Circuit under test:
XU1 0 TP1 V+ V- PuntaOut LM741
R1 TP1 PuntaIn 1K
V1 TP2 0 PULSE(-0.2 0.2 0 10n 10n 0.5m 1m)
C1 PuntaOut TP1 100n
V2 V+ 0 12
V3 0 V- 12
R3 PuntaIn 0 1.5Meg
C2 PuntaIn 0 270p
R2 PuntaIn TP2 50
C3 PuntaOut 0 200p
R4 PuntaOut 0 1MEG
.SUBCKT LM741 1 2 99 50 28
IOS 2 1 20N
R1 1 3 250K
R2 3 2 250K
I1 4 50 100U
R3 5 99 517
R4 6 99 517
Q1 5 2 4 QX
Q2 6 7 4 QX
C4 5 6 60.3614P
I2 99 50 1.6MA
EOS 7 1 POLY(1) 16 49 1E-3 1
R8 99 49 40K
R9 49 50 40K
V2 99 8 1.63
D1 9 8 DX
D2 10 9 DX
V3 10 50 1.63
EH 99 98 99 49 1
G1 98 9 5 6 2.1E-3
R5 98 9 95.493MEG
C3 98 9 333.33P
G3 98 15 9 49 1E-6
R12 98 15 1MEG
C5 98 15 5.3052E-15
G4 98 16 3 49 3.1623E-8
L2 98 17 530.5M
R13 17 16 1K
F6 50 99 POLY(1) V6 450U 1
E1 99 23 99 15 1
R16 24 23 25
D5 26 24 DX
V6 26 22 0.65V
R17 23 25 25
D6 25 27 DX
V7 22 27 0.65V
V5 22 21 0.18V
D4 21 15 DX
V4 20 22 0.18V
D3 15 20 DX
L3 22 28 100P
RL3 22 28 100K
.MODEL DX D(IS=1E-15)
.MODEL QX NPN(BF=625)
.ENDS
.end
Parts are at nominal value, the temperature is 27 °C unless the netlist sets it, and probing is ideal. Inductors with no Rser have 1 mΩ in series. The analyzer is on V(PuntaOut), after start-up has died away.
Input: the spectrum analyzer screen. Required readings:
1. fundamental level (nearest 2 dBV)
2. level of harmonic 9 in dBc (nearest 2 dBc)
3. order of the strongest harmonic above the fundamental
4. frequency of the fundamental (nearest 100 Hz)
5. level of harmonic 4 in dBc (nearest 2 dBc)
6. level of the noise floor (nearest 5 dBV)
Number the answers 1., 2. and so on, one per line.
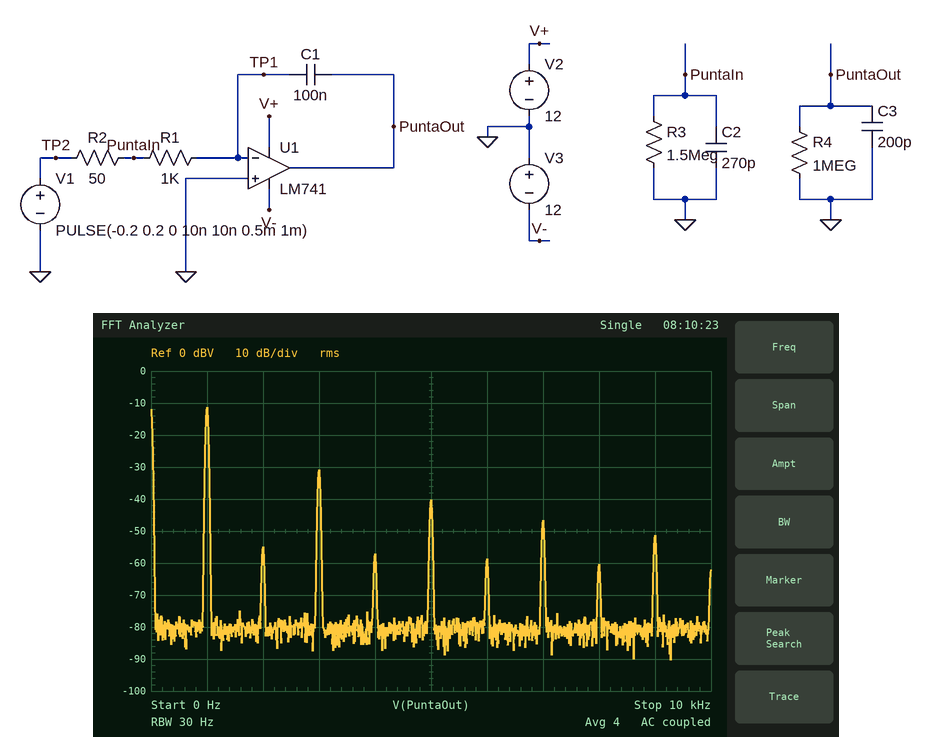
1. -12 dBV
2. -40 dBc
3. 3
4. 1.0 kHz
5. -46 dBc
6. -80 dBV
